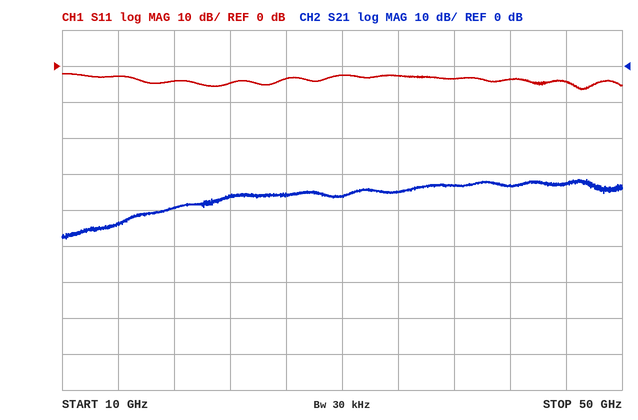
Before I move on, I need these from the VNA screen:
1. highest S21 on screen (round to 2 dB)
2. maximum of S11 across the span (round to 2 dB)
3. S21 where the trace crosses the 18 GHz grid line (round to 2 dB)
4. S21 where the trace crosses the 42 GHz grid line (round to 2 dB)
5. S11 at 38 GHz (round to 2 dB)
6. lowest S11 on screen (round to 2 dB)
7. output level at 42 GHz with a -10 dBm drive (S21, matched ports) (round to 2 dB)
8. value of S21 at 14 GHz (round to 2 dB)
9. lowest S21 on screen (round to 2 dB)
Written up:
-32 dB
-2 dB
-40 dB
-34 dB
-4 dB
-6 dB
-44 dBm
-44 dB
-48 dB
